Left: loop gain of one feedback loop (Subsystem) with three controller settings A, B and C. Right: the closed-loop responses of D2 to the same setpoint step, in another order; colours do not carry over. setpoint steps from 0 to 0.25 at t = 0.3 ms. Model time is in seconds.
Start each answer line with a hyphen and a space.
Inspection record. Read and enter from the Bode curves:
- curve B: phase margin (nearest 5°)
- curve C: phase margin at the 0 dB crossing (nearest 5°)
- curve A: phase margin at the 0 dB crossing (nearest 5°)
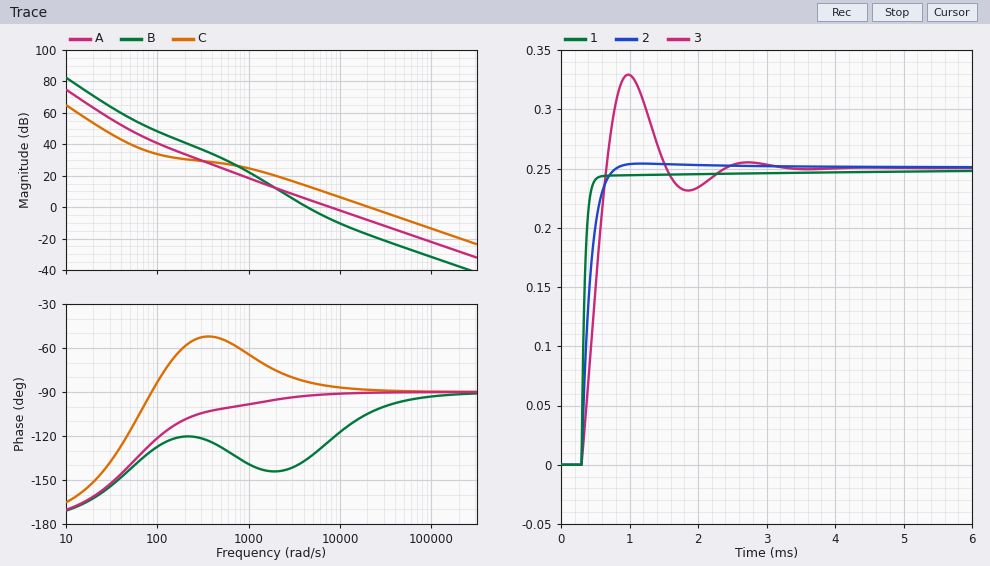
- 45°
- 90°
- 90°
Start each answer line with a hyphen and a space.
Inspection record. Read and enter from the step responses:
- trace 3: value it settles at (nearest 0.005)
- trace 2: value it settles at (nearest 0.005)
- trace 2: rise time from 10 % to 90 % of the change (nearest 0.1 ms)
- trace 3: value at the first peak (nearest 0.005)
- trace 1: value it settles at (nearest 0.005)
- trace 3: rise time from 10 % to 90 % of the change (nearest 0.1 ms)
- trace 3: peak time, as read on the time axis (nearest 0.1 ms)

- 0.250
- 0.250
- 0.3 ms
- 0.330
- 0.250
- 0.3 ms
- 1.0 ms
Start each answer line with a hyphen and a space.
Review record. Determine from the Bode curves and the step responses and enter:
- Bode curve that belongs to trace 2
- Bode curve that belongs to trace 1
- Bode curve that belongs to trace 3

- A
- C
- B
